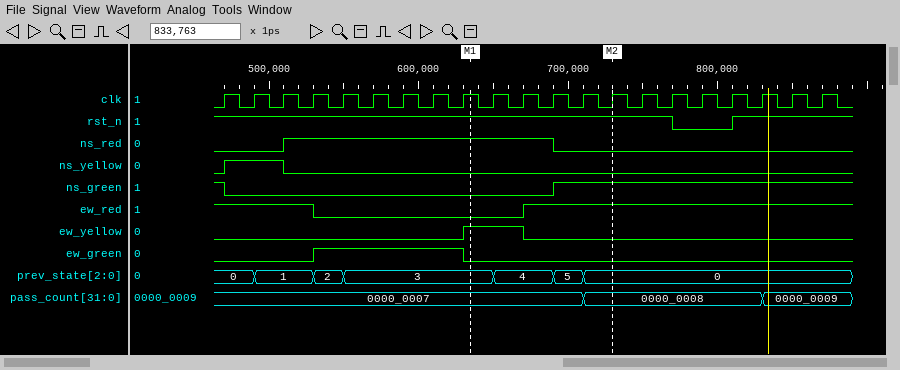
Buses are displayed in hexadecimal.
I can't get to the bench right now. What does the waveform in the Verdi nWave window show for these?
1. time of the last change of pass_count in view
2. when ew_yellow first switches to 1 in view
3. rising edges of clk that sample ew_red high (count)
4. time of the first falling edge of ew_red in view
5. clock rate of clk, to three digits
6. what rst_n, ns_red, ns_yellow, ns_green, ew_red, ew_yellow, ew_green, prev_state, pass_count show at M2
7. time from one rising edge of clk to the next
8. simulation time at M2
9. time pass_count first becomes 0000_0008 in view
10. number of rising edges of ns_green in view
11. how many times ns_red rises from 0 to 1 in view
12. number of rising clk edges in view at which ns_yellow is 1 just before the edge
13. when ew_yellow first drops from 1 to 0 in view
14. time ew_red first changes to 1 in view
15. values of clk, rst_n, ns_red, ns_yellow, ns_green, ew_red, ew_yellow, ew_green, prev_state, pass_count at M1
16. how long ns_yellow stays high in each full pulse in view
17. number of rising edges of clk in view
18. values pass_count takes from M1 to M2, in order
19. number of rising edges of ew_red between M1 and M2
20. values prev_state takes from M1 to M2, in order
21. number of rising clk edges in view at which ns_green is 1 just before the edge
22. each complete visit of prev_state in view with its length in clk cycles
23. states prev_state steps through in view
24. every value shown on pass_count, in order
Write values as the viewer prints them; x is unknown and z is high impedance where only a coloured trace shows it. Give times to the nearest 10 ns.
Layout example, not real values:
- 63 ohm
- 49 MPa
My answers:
- 830 ns
- 630 ns
- 14
- 530 ns
- 50.0 MHz
- rst_n=1, ns_red=0, ns_yellow=0, ns_green=1, ew_red=1, ew_yellow=0, ew_green=0, prev_state=0, pass_count=0000_0008
- 20 ns
- 730 ns
- 710 ns
- 1
- 1
- 2
- 670 ns
- 670 ns
- clk=1, rst_n=1, ns_red=1, ns_yellow=0, ns_green=0, ew_red=0, ew_yellow=1, ew_green=0, prev_state=3, pass_count=0000_0007
- 40 ns
- 21
- 0000_0007, 0000_0008
- 1
- 3, 4, 5, 0
- 10
- 1: 2, 2: 1, 3: 5, 4: 2, 5: 1
- 0, 1, 2, 3, 4, 5, 0
- 0000_0007, 0000_0008, 0000_0009
